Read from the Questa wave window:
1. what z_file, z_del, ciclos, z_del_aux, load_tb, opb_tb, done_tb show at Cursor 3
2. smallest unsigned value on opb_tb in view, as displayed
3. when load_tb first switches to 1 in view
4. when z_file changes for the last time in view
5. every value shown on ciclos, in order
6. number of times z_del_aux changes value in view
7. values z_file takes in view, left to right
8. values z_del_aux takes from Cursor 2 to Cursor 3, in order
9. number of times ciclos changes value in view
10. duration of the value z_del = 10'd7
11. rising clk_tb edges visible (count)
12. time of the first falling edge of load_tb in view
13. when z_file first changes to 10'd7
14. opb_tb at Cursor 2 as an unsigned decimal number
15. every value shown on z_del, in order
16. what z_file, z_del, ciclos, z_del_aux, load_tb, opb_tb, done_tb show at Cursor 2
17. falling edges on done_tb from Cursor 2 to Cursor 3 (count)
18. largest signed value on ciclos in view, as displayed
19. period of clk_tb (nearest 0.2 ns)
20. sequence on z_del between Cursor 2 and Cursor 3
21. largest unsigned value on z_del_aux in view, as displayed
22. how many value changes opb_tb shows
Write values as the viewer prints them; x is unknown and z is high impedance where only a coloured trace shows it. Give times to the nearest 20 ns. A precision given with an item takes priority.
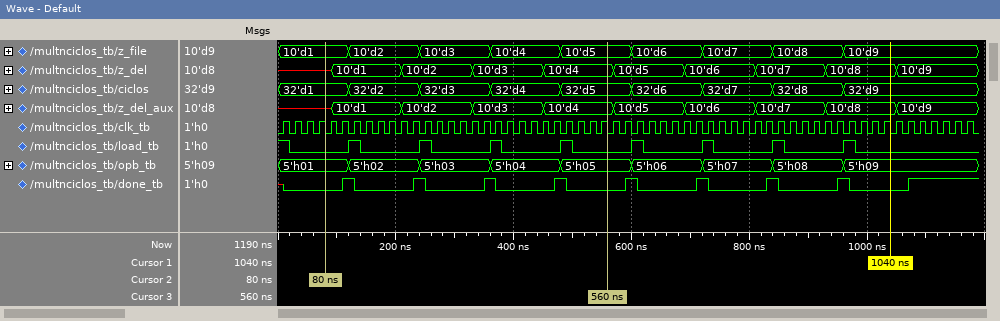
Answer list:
z_file=10'd5, z_del=10'd4, ciclos=32'd5, z_del_aux=10'd4, load_tb=0, opb_tb=5'h05, done_tb=0
5'h01
120 ns
960 ns
32'd1, 32'd2, 32'd3, 32'd4, 32'd5, 32'd6, 32'd7, 32'd8, 32'd9
9
10'd1, 10'd2, 10'd3, 10'd4, 10'd5, 10'd6, 10'd7, 10'd8, 10'd9
x, 10'd1, 10'd2, 10'd3, 10'd4
8
120 ns
59
20 ns
720 ns
1
x, 10'd1, 10'd2, 10'd3, 10'd4, 10'd5, 10'd6, 10'd7, 10'd8, 10'd9
z_file=10'd1, z_del=x, ciclos=32'd1, z_del_aux=x, load_tb=0, opb_tb=5'h01, done_tb=0
4
32'd9
20 ns
x, 10'd1, 10'd2, 10'd3, 10'd4
10'd9
8
